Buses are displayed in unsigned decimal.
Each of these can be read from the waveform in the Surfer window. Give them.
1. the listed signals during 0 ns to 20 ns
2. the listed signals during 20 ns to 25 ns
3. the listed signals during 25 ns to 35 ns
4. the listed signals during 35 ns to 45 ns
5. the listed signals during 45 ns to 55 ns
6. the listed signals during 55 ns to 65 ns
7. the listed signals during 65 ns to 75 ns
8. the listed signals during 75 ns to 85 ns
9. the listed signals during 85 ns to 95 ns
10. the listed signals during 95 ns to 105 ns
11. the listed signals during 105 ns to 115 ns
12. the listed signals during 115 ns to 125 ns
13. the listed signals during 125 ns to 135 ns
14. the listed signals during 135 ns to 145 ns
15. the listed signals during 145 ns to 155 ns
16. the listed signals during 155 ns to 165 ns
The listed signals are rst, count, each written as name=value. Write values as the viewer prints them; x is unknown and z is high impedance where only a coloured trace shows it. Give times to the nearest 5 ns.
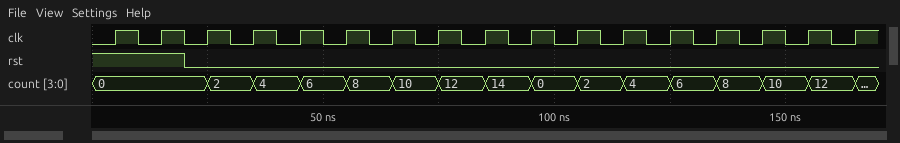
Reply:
rst=1, count=0
rst=0, count=0
rst=0, count=2
rst=0, count=4
rst=0, count=6
rst=0, count=8
rst=0, count=10
rst=0, count=12
rst=0, count=14
rst=0, count=0
rst=0, count=2
rst=0, count=4
rst=0, count=6
rst=0, count=8
rst=0, count=10
rst=0, count=12
